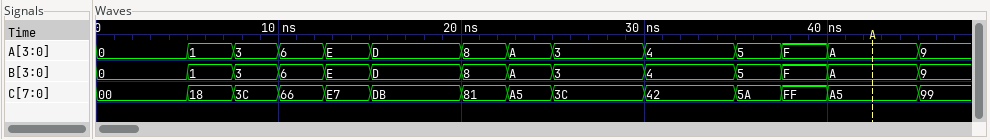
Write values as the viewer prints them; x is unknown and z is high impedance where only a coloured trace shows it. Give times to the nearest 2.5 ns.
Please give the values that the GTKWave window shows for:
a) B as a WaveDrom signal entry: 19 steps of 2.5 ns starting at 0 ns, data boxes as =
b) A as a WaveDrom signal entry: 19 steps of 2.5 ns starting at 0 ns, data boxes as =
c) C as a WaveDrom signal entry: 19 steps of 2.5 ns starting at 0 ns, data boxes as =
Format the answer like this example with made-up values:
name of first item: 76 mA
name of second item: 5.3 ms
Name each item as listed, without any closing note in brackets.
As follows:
B as a WaveDrom signal entry: 19 steps of 2.5 ns starting at 0 ns, data boxes as =: {name: 'B', wave: '=.=====.===.=.===.=', data: '0 1 3 6 E D 8 A 3 4 5 F A 9'}
A as a WaveDrom signal entry: 19 steps of 2.5 ns starting at 0 ns, data boxes as =: {name: 'A', wave: '=.=====.===.=.===.=', data: '0 1 3 6 E D 8 A 3 4 5 F A 9'}
C as a WaveDrom signal entry: 19 steps of 2.5 ns starting at 0 ns, data boxes as =: {name: 'C', wave: '=.=====.===.=.===.=', data: '00 18 3C 66 E7 DB 81 A5 3C 42 5A FF A5 99'}
